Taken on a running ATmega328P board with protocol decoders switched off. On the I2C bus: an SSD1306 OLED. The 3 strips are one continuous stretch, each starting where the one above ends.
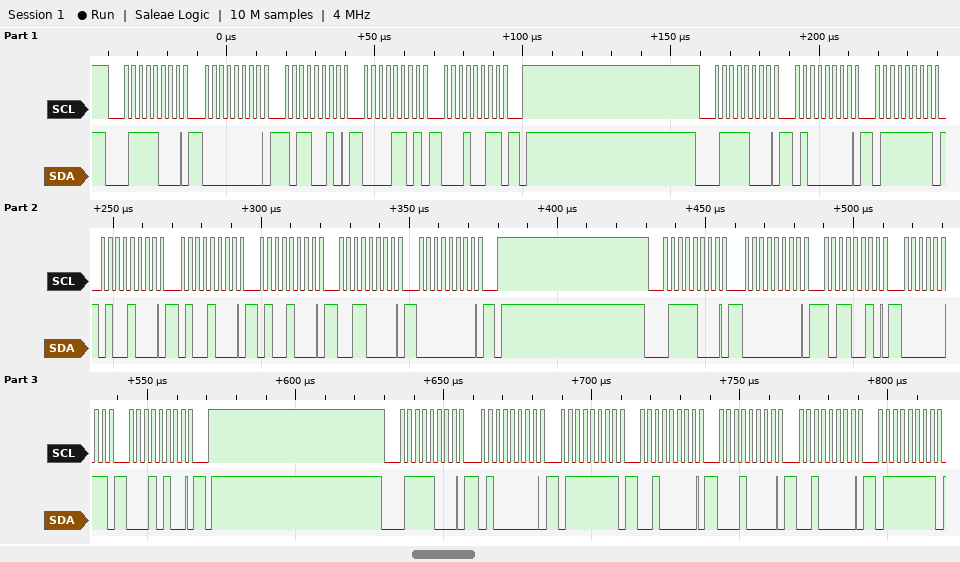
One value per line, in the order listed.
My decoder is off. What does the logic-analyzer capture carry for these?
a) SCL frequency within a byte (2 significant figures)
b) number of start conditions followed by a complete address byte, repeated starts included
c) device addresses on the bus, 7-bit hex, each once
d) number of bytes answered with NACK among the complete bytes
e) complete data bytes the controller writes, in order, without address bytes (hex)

400 kHz
4
0x3C
0
00 B2 0D 13 40 7F 48 48 48 30 00 00 B2 03 14 40 7F 20 10 20 7F
